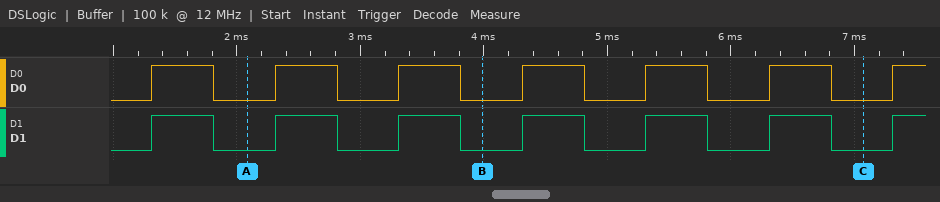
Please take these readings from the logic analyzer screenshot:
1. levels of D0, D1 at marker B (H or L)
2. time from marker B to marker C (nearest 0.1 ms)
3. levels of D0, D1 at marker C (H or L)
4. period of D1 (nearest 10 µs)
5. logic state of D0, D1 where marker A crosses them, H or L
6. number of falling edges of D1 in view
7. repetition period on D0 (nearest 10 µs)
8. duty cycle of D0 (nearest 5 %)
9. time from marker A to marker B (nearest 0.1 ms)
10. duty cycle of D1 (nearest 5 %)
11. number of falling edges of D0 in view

D0=L, D1=L
3.1 ms
D0=L, D1=L
1000 µs
D0=L, D1=L
6
1000 µs
50 %
1.9 ms
50 %
6
